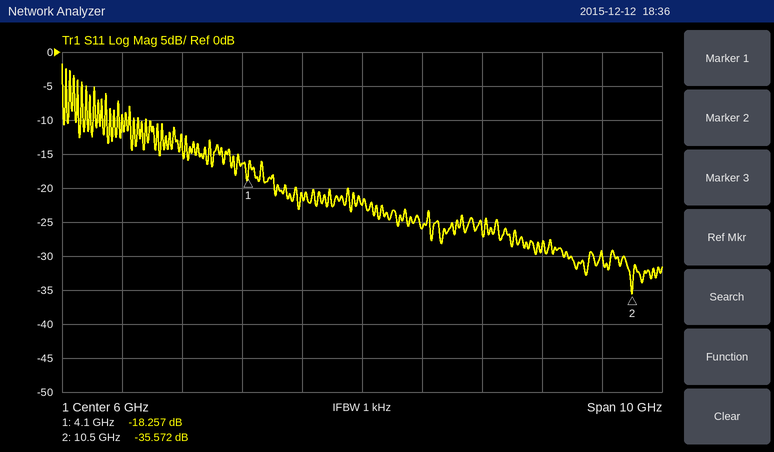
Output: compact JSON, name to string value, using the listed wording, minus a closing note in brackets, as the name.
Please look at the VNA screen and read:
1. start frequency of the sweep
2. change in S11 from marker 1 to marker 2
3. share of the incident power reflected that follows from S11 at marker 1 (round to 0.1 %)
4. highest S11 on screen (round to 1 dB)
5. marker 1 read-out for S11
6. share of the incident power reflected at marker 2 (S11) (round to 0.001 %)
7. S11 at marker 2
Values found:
{"start frequency of the sweep": "1 GHz", "change in S11 from marker 1 to marker 2": "-17.315 dB", "share of the incident power reflected that follows from S11 at marker 1": "1.5 %", "highest S11 on screen": "-2 dB", "marker 1 read-out for S11": "-18.257 dB", "share of the incident power reflected at marker 2 (S11)": "0.028 %", "S11 at marker 2": "-35.572 dB"}
